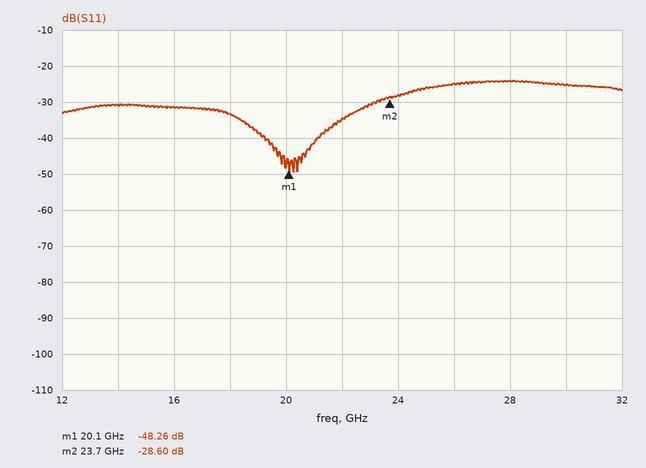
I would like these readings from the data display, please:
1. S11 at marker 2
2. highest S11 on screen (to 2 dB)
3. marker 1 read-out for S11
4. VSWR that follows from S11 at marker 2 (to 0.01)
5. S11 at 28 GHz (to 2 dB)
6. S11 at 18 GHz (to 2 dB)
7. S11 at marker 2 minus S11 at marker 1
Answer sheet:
-28.60 dB
-24 dB
-48.26 dB
1.08
-24 dB
-34 dB
19.66 dB
